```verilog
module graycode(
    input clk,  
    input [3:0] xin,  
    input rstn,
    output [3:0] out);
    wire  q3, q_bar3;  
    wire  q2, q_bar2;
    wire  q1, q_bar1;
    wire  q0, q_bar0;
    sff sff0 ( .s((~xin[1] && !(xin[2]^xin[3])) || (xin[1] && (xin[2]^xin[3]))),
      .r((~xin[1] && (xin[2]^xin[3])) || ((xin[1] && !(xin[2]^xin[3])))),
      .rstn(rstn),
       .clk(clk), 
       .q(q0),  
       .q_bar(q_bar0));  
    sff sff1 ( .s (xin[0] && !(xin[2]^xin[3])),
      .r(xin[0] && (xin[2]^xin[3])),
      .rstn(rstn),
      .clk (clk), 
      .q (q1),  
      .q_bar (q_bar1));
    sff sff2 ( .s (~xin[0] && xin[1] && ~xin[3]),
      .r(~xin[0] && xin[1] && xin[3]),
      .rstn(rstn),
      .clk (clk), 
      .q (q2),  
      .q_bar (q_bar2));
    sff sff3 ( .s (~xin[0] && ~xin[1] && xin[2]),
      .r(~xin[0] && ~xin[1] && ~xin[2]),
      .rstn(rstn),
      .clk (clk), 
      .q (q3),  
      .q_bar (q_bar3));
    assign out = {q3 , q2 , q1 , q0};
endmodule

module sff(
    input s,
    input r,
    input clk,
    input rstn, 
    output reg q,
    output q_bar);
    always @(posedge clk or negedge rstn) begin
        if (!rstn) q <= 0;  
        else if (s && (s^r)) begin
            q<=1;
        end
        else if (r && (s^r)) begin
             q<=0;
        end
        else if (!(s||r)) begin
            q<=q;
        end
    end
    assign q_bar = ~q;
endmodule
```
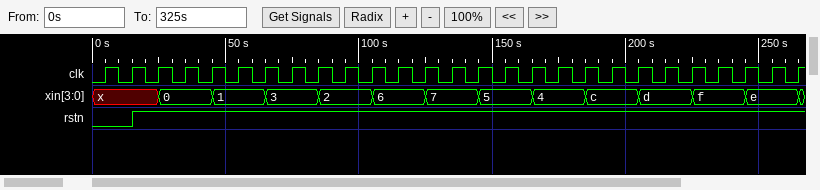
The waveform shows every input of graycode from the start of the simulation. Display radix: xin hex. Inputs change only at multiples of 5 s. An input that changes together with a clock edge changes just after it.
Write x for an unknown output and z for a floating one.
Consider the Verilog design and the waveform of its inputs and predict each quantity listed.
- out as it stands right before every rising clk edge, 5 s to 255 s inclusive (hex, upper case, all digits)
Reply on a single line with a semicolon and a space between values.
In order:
0, 0, 0, 0, 1, 1, 3, 3, 2, 2, 6, 6, 7, 7, 5, 5, 4, 4, C, C, D, D, F, F, E, E
